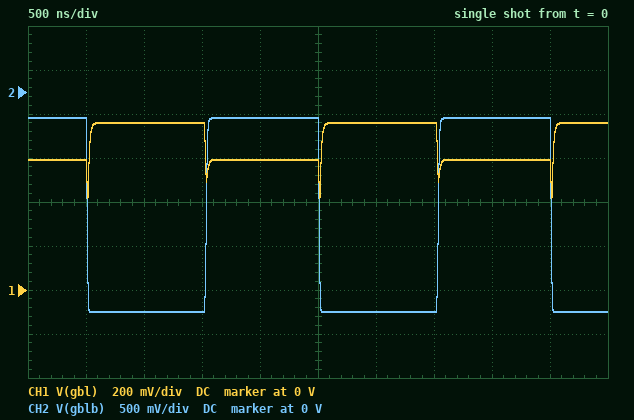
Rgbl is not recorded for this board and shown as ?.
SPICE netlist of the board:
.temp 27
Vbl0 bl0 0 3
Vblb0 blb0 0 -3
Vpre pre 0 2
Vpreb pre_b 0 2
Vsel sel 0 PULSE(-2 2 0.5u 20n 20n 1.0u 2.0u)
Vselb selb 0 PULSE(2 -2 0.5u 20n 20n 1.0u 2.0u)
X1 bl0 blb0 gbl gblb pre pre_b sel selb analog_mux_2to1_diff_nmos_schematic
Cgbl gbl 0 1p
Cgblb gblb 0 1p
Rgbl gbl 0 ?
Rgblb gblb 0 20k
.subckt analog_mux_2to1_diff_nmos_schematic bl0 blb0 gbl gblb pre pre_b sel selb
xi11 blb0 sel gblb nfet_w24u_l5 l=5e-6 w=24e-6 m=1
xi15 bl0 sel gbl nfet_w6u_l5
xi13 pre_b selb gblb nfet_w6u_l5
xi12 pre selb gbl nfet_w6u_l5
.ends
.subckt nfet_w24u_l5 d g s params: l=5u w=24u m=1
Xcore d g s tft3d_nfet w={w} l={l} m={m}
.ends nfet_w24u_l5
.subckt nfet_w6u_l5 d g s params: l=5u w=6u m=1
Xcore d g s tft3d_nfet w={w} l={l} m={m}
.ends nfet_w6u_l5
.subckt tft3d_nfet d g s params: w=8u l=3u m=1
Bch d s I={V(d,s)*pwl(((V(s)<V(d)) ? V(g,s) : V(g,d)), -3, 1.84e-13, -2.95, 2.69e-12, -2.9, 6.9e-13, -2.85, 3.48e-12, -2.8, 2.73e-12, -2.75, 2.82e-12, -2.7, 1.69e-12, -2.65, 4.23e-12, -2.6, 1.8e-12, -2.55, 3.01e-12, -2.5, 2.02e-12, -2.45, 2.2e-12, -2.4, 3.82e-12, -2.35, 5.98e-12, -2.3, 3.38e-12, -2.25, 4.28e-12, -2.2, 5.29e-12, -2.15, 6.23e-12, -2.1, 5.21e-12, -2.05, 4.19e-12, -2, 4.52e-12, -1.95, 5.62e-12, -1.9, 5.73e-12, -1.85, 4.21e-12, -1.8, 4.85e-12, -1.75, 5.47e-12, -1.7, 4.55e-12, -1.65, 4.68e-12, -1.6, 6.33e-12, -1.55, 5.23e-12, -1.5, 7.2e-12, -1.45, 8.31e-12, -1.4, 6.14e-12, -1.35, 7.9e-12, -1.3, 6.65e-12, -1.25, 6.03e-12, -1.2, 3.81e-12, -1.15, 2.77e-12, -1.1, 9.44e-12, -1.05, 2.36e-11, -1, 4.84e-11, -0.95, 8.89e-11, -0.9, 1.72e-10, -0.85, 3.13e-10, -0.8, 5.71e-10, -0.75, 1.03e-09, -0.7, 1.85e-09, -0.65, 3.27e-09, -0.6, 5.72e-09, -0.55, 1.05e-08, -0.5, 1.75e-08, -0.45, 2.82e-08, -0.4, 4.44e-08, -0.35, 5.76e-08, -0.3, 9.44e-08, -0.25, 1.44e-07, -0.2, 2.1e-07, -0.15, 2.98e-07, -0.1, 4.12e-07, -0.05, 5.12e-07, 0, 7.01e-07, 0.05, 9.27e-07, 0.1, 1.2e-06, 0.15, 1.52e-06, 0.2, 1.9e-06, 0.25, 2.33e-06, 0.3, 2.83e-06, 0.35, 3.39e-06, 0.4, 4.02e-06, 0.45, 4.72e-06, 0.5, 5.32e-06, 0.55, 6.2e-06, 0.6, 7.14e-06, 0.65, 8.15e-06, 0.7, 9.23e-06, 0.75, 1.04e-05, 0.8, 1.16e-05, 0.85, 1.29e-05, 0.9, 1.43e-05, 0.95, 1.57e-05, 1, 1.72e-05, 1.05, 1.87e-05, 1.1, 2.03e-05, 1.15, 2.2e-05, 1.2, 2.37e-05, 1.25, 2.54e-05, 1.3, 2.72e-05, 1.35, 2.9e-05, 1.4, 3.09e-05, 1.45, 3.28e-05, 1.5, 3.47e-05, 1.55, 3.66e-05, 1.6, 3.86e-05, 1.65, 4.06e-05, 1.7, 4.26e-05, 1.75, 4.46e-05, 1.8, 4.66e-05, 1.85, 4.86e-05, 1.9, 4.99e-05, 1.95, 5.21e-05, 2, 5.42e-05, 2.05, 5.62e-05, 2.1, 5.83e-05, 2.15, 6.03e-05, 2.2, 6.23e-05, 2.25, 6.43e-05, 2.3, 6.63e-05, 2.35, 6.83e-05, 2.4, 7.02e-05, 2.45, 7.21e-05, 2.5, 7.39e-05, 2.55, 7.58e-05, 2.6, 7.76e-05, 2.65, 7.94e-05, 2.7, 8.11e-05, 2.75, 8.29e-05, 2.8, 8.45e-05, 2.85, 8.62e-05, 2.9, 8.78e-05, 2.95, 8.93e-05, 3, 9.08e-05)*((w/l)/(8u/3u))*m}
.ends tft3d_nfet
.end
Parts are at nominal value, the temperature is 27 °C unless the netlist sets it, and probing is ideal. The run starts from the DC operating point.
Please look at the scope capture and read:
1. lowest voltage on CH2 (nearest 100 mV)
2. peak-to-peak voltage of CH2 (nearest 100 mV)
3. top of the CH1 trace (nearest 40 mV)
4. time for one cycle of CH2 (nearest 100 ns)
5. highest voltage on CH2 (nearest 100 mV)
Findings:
-2.5 V
2.2 V
760 mV
2.0 µs
-300 mV
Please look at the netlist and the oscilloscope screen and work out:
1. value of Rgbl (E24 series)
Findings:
30 kΩ
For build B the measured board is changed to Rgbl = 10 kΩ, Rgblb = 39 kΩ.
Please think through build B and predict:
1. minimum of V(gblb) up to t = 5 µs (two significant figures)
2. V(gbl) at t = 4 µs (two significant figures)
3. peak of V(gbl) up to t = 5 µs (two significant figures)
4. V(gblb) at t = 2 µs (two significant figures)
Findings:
-2.7 V
320 mV
430 mV
-360 mV
